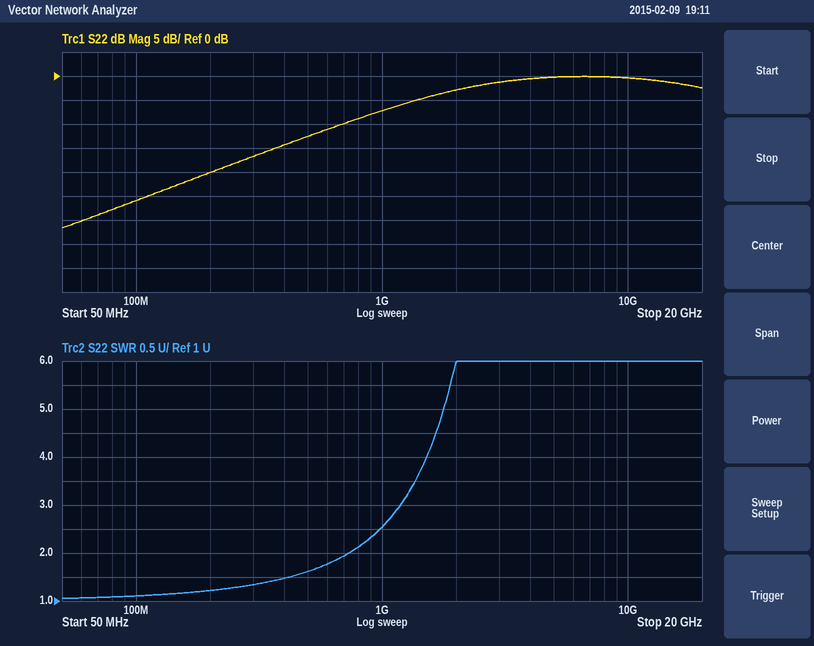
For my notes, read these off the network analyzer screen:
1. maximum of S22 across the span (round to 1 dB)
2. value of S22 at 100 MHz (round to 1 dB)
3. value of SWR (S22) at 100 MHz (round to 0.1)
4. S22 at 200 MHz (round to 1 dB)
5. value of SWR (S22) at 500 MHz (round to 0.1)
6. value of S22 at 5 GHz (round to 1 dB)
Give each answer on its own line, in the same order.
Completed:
0 dB
-26 dB
1.1
-20 dB
1.6
0 dB
